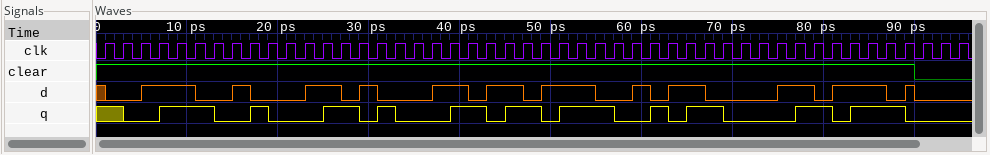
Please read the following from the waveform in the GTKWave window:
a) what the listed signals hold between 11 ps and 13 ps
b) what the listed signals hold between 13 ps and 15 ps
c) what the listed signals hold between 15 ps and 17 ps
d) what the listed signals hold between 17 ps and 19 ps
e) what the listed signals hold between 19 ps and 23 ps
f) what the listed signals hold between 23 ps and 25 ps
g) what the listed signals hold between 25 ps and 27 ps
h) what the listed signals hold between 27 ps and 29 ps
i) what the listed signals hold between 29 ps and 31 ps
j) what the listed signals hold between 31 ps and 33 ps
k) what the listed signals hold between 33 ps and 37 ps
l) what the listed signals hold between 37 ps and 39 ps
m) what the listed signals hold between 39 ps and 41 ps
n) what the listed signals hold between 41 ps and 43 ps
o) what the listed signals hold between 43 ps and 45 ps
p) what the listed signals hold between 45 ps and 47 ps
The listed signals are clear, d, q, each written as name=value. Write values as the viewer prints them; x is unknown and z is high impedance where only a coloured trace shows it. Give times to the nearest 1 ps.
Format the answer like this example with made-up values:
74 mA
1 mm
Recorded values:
clear=1, d=0, q=1
clear=1, d=0, q=0
clear=1, d=1, q=0
clear=1, d=0, q=1
clear=1, d=0, q=0
clear=1, d=1, q=0
clear=1, d=1, q=1
clear=1, d=0, q=1
clear=1, d=1, q=0
clear=1, d=0, q=1
clear=1, d=0, q=0
clear=1, d=1, q=0
clear=1, d=1, q=1
clear=1, d=0, q=1
clear=1, d=1, q=0
clear=1, d=1, q=1
